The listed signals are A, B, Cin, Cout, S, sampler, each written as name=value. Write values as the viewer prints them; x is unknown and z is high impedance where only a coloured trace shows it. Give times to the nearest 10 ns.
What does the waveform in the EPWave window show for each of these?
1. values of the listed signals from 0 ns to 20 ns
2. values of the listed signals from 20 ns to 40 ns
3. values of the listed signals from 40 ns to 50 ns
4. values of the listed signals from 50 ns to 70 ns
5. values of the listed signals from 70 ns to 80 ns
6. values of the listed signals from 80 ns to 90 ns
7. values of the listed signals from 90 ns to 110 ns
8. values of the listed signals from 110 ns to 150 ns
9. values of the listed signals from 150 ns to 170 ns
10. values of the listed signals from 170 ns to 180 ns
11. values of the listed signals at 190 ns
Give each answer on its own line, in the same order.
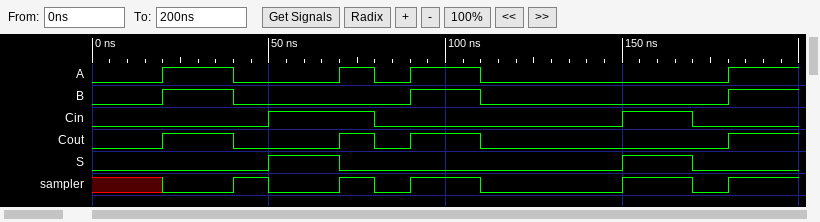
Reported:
A=0, B=0, Cin=0, Cout=0, S=0, sampler=x
A=1, B=1, Cin=0, Cout=1, S=0, sampler=0
A=0, B=0, Cin=0, Cout=0, S=0, sampler=1
A=0, B=0, Cin=1, Cout=0, S=1, sampler=0
A=1, B=0, Cin=1, Cout=1, S=0, sampler=1
A=0, B=0, Cin=0, Cout=0, S=0, sampler=0
A=1, B=1, Cin=0, Cout=1, S=0, sampler=1
A=0, B=0, Cin=0, Cout=0, S=0, sampler=0
A=0, B=0, Cin=1, Cout=0, S=1, sampler=1
A=0, B=0, Cin=0, Cout=0, S=0, sampler=0
A=1, B=1, Cin=0, Cout=1, S=0, sampler=1
